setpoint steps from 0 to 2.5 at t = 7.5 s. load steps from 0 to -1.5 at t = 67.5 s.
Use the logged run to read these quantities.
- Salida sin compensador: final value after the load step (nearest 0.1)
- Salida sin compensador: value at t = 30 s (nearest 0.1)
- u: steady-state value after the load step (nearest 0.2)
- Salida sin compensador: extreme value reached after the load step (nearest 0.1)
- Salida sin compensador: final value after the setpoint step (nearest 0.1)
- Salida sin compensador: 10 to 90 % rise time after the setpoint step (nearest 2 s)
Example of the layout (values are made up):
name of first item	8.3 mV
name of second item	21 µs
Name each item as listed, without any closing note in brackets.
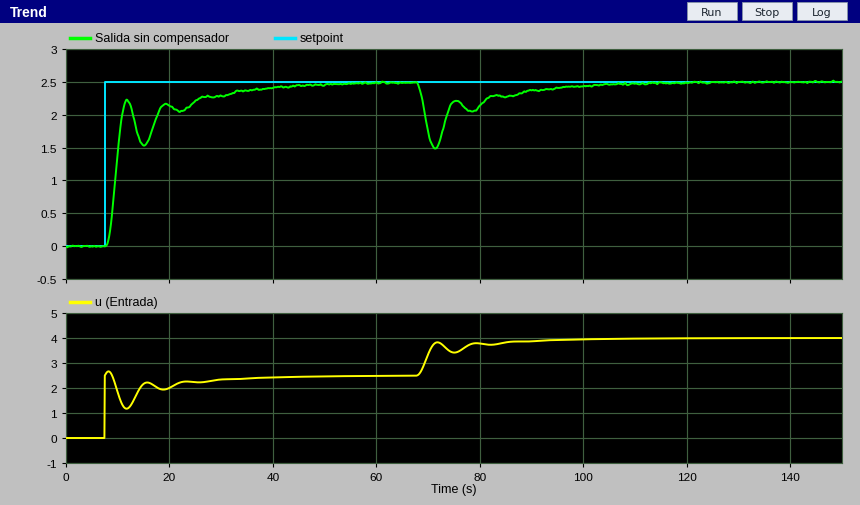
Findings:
Salida sin compensador: final value after the load step	2.5
Salida sin compensador: value at t = 30 s	2.3
u: steady-state value after the load step	4.0
Salida sin compensador: extreme value reached after the load step	1.5
Salida sin compensador: final value after the setpoint step	2.5
Salida sin compensador: 10 to 90 % rise time after the setpoint step	18 s
